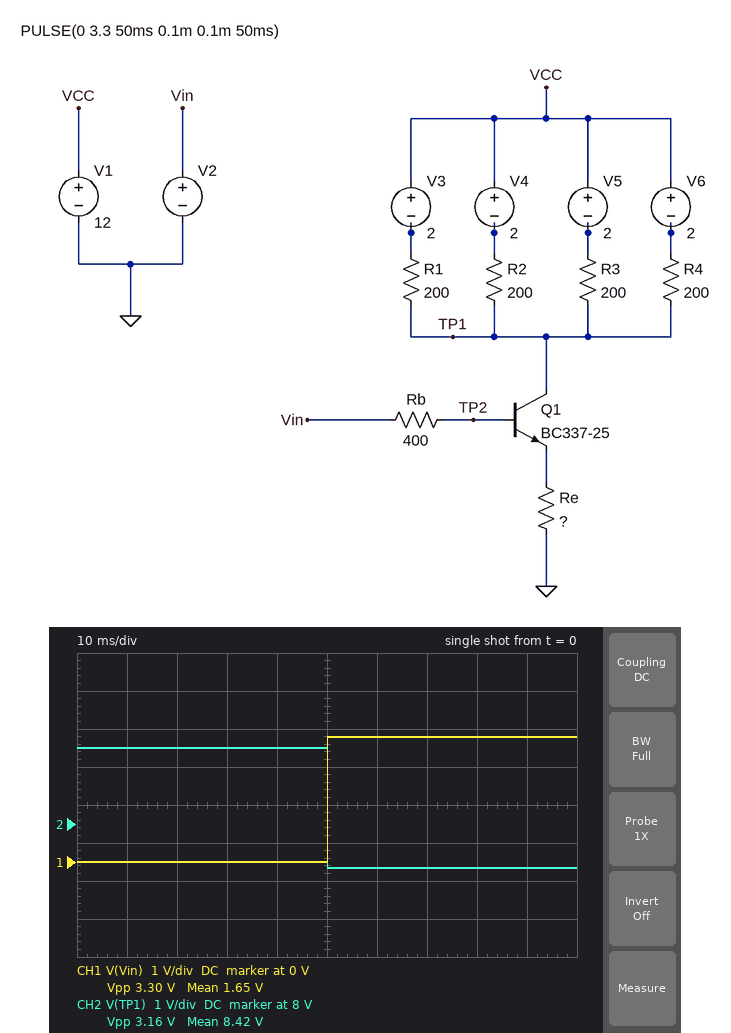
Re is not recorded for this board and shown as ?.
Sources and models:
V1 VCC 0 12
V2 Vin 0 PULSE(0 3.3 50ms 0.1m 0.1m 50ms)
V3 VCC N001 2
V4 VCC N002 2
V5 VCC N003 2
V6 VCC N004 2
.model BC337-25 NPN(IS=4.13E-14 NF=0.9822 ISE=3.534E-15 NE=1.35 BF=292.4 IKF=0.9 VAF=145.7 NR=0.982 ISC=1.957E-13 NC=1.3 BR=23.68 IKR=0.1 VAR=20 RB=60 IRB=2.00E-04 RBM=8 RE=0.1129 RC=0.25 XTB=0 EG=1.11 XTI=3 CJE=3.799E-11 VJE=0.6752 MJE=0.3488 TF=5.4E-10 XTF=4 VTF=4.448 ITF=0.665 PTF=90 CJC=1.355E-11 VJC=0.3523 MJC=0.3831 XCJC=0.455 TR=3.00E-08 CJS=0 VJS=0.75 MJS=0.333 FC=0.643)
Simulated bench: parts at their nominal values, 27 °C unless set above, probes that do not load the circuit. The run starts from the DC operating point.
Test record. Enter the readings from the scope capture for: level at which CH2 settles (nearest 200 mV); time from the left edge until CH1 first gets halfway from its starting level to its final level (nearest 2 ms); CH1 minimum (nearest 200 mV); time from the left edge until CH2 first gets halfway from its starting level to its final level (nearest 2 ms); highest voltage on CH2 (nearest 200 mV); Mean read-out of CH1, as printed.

6.8 V
50 ms
0 V
50 ms
10.0 V
1.65 V
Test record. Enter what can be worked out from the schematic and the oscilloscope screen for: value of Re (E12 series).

39 Ω
